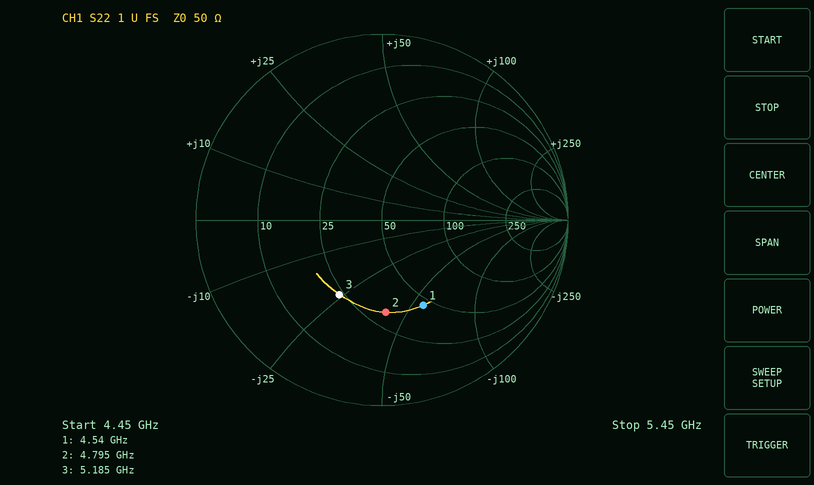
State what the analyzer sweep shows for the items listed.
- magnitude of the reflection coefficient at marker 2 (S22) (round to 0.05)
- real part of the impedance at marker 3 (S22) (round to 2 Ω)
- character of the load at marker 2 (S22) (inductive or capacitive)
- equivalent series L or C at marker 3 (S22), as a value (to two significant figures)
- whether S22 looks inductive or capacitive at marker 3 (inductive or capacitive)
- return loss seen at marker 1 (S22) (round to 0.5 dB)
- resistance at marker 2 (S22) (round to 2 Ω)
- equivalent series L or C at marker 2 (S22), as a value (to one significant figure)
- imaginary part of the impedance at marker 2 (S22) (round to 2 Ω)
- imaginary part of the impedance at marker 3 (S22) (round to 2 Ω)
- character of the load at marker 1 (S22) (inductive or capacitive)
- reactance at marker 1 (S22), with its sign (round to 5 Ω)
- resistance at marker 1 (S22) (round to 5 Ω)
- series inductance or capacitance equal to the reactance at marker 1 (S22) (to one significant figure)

0.50
24 Ω
capacitive
1.3 pF
capacitive
6.0 dB
32 Ω
800 fF
-42 Ω
-24 Ω
capacitive
-55 Ω
45 Ω
600 fF
